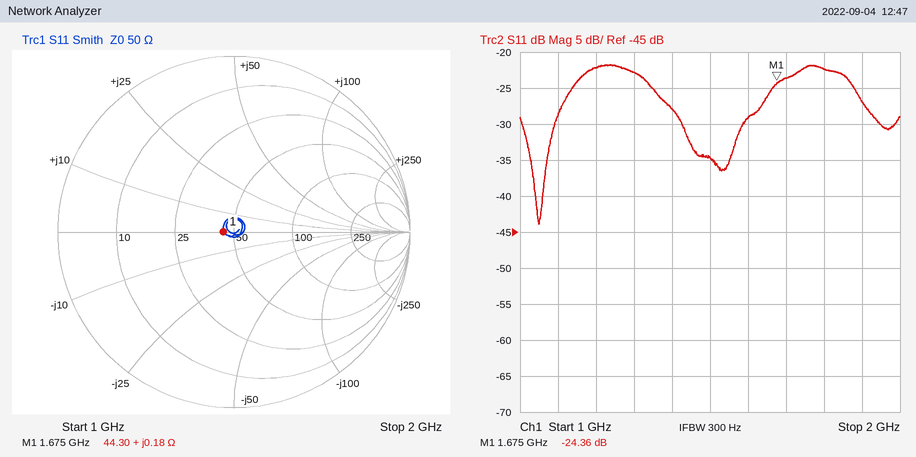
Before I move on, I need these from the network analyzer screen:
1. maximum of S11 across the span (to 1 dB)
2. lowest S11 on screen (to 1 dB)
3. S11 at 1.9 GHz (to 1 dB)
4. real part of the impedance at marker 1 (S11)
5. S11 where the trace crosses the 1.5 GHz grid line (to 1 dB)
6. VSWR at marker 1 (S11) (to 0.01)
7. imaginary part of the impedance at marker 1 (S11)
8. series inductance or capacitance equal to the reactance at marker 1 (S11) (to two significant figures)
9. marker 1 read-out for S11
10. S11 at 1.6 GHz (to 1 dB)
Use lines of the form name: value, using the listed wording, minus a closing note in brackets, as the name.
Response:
maximum of S11 across the span: -22 dB
lowest S11 on screen: -44 dB
S11 at 1.9 GHz: -27 dB
real part of the impedance at marker 1: 44.30 Ω
S11 where the trace crosses the 1.5 GHz grid line: -35 dB
VSWR at marker 1 (S11): 1.13
imaginary part of the impedance at marker 1: +0.18 Ω
series inductance or capacitance equal to the reactance at marker 1 (S11): 17 pH
marker 1 read-out for S11: -24.36 dB
S11 at 1.6 GHz: -29 dB
